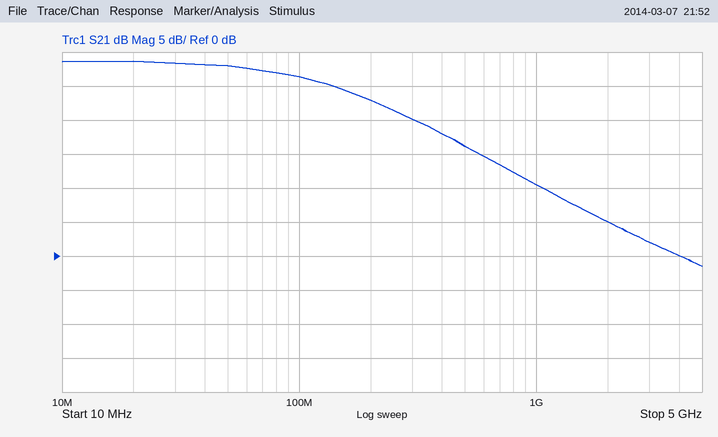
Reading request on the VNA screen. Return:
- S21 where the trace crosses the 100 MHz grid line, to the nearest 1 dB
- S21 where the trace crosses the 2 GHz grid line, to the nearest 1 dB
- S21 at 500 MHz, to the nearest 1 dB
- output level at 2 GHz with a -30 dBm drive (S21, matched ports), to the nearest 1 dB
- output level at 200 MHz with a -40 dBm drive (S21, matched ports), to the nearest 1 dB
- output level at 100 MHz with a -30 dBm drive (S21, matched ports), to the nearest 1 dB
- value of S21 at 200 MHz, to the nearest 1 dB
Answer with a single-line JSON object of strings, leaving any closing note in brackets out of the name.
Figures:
{"S21 where the trace crosses the 100 MHz grid line, to the nearest 1 dB": "26 dB", "S21 where the trace crosses the 2 GHz grid line, to the nearest 1 dB": "5 dB", "S21 at 500 MHz, to the nearest 1 dB": "16 dB", "output level at 2 GHz with a -30 dBm drive (S21, matched ports), to the nearest 1 dB": "-25 dBm", "output level at 200 MHz with a -40 dBm drive (S21, matched ports), to the nearest 1 dB": "-17 dBm", "output level at 100 MHz with a -30 dBm drive (S21, matched ports), to the nearest 1 dB": "-4 dBm", "value of S21 at 200 MHz, to the nearest 1 dB": "23 dB"}
